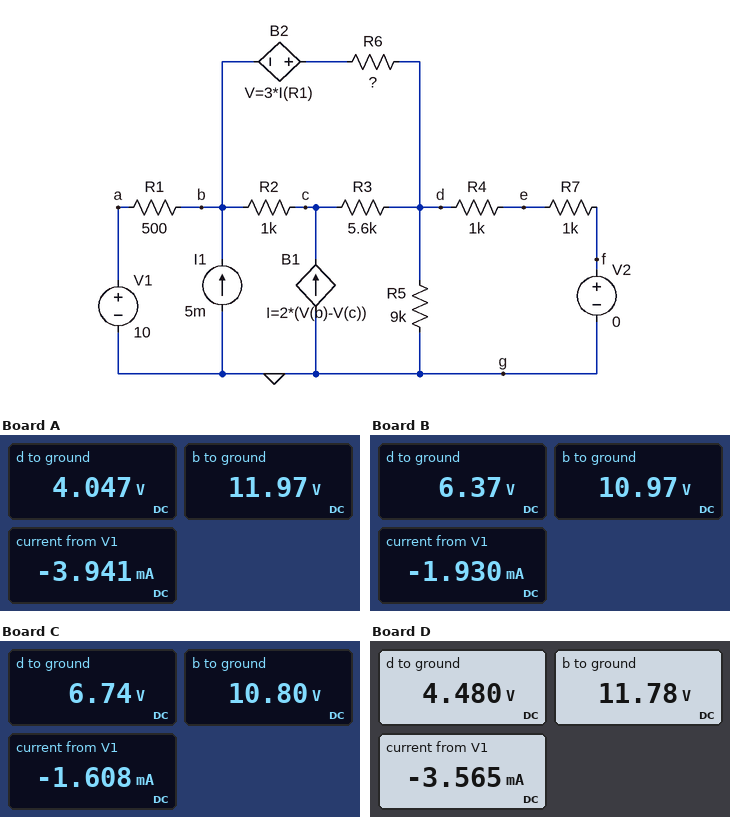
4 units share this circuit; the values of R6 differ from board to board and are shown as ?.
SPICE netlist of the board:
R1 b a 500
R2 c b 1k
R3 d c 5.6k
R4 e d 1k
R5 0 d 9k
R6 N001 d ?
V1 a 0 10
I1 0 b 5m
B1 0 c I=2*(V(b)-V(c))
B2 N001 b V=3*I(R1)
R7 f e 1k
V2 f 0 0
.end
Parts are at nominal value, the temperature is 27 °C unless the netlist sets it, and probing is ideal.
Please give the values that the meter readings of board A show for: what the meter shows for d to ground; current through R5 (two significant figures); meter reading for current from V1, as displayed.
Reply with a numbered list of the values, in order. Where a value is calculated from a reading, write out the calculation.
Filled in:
1. 4.047 V
2. (4.047 V) / 9 kΩ = 450 µA
3. -3.941 mA
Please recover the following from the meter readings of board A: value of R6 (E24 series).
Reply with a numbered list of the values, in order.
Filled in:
1. 7.5 kΩ
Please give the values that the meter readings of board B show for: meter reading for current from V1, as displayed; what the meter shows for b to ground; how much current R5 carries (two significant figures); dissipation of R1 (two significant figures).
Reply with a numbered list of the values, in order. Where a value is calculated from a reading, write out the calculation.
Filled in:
1. -1.930 mA
2. 10.97 V
3. (6.37 V) / 9 kΩ = 710 µA
4. (10.97 V - 10 V)^2 / 500 Ω = 1.9 mW
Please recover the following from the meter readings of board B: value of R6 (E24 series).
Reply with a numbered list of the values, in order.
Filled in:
1. 1.5 kΩ
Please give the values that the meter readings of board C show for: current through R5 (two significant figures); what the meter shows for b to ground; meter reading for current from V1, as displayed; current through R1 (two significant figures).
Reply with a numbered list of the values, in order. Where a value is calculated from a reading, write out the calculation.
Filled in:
1. (6.74 V) / 9 kΩ = 750 µA
2. 10.80 V
3. -1.608 mA
4. (10.8 V - 10 V) / 500 Ω = 1.6 mA
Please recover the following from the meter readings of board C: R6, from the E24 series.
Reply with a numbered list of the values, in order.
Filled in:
1. 1.2 kΩ
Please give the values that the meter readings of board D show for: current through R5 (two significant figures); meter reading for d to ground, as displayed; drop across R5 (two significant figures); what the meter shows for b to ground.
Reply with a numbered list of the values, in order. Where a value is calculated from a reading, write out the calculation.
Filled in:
1. (4.48 V) / 9 kΩ = 500 µA
2. 4.480 V
3. 4.48 V = 4.5 V
4. 11.78 V
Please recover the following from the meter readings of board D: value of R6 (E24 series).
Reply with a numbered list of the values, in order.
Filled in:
1. 5.1 kΩ
